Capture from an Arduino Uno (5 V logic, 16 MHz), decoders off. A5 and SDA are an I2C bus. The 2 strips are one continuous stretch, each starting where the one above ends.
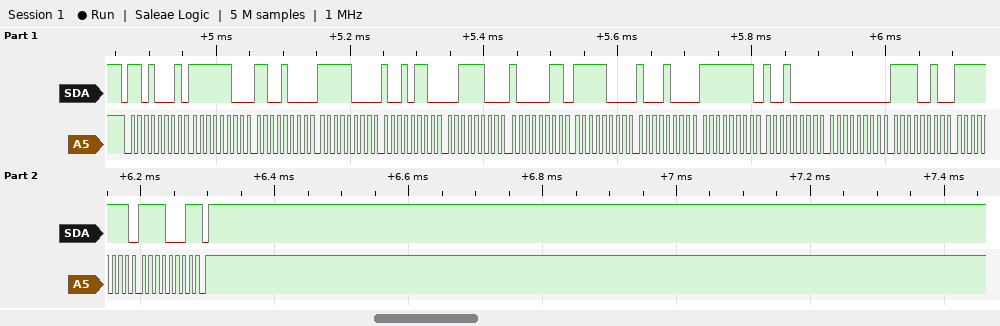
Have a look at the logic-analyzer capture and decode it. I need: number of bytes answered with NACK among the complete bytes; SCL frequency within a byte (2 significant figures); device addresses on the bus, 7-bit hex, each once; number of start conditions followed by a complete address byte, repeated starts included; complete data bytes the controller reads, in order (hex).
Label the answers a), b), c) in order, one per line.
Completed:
a) 1
b) 100 kHz
c) 0x68
d) 1
e) FC C8 F8 96 3C 83 F8 88 FF 90 00 F2 FF F1
